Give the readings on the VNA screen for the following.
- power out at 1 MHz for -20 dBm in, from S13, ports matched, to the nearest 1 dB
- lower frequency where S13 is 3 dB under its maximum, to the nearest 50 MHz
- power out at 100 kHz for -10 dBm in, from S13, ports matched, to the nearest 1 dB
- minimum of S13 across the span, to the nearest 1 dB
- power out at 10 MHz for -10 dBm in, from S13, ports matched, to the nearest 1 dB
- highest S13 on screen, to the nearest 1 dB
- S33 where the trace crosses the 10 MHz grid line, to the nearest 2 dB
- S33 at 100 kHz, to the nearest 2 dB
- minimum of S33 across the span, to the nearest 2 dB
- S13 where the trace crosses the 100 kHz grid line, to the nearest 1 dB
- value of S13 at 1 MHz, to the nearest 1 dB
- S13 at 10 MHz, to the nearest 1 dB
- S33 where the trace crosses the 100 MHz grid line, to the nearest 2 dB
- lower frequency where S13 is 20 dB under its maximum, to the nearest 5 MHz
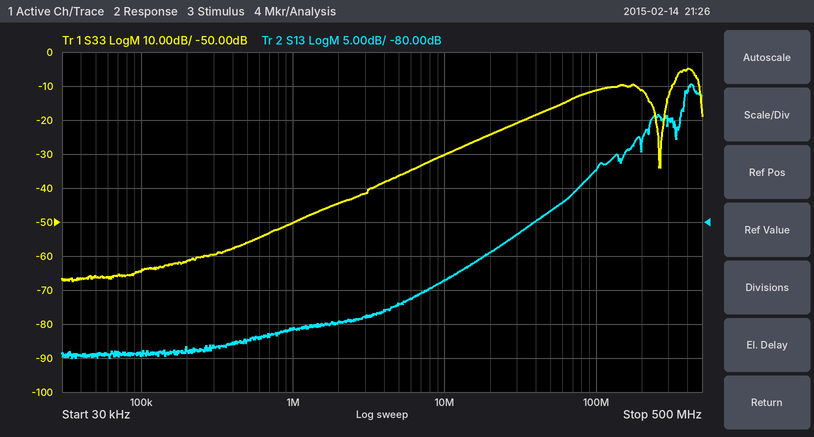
-116 dBm
400 MHz
-109 dBm
-100 dB
-99 dBm
-60 dB
-30 dB
-64 dB
-68 dB
-99 dB
-96 dB
-89 dB
-12 dB
40 MHz
